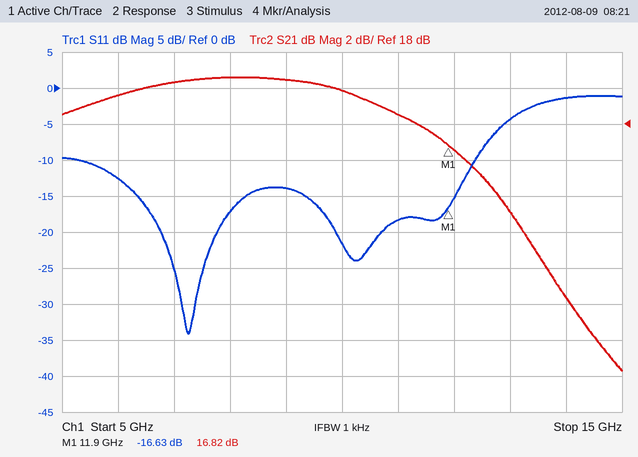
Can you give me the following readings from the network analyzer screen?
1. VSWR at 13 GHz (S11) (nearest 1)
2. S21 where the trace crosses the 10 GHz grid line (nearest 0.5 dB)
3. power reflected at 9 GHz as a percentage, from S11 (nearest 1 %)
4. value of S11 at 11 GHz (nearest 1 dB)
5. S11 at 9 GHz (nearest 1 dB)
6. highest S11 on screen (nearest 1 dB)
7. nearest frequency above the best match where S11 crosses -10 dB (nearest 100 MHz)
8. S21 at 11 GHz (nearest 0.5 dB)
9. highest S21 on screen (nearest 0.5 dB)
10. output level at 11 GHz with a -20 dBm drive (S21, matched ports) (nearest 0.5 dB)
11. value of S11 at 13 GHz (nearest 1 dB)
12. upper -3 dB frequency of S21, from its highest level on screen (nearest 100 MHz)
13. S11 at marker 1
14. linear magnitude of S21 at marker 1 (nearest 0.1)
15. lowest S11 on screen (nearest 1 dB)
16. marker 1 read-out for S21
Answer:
4
20.0 dB
4 %
-18 dB
-14 dB
-1 dB
12.4 GHz
18.5 dB
20.5 dB
-1.5 dBm
-4 dB
11.6 GHz
-16.63 dB
6.9
-34 dB
16.82 dB
